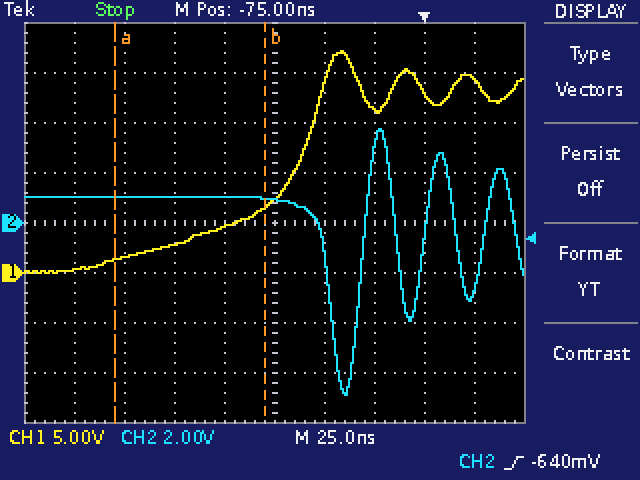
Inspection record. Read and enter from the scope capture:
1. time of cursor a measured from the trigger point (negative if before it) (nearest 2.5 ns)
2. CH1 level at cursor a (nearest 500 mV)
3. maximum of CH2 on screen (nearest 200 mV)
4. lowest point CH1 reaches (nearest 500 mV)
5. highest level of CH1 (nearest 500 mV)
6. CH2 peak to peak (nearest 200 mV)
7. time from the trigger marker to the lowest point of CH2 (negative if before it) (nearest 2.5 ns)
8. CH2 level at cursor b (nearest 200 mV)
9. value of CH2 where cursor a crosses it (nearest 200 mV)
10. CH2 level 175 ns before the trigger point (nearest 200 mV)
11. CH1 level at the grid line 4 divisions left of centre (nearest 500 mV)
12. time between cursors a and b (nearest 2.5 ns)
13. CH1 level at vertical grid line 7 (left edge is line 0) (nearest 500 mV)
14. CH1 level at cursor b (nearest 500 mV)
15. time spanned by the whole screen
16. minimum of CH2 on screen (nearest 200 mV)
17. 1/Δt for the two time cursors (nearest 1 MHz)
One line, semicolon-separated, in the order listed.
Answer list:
-155.0 ns; 1.5 V; 3.8 V; 0.0 V; 22.0 V; 10.6 V; -40.0 ns; 1.0 V; 1.0 V; 1.0 V; 500 mV; 75.0 ns; 16.5 V; 6.5 V; 250 ns; -6.8 V; 13 MHz
